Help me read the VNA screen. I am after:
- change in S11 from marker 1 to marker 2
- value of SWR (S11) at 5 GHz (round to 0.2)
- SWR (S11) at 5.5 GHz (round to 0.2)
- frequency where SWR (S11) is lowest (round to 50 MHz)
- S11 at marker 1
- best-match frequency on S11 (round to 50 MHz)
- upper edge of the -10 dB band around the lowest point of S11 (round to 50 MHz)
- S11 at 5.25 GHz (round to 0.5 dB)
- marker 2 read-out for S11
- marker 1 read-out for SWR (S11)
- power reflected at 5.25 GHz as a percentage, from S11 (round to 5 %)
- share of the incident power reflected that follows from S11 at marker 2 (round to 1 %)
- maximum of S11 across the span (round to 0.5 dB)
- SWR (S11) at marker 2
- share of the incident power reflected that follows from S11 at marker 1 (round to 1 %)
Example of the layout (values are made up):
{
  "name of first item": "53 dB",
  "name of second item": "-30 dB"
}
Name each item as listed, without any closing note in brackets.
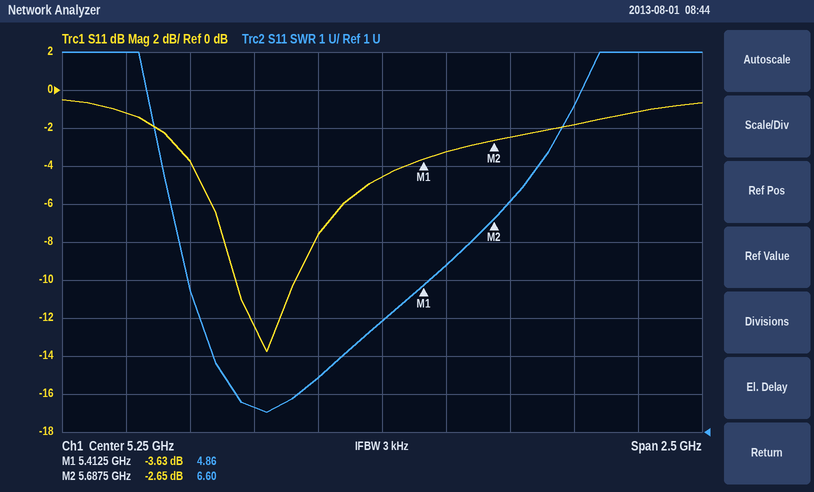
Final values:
{
  "change in S11 from marker 1 to marker 2": "0.98 dB",
  "value of SWR (S11) at 5 GHz": "2.4",
  "SWR (S11) at 5.5 GHz": "5.4",
  "frequency where SWR (S11) is lowest": "4.80 GHz",
  "S11 at marker 1": "-3.63 dB",
  "best-match frequency on S11": "4.80 GHz",
  "upper edge of the -10 dB band around the lowest point of S11": "4.90 GHz",
  "S11 at 5.25 GHz": "-4.5 dB",
  "marker 2 read-out for S11": "-2.65 dB",
  "marker 1 read-out for SWR": "4.86",
  "power reflected at 5.25 GHz as a percentage, from S11": "35 %",
  "share of the incident power reflected that follows from S11 at marker 2": "54 %",
  "maximum of S11 across the span": "-0.5 dB",
  "SWR (S11) at marker 2": "6.60",
  "share of the incident power reflected that follows from S11 at marker 1": "43 %"
}
